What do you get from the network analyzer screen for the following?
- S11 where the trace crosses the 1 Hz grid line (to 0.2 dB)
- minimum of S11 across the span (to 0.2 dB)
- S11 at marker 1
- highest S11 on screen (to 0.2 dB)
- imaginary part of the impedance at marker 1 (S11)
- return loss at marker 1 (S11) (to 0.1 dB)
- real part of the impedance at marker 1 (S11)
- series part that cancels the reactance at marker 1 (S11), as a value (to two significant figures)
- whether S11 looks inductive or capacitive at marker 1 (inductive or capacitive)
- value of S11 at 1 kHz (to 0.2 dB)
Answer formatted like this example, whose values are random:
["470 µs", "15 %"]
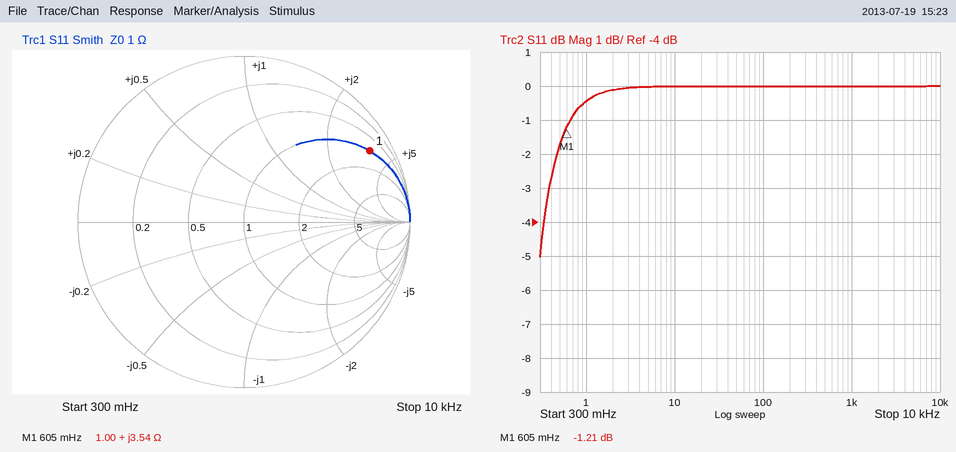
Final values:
["-0.4 dB", "-5.0 dB", "-1.21 dB", "0.0 dB", "+3.54 Ω", "1.2 dB", "1.00 Ω", "74 mF", "inductive", "0.0 dB"]
